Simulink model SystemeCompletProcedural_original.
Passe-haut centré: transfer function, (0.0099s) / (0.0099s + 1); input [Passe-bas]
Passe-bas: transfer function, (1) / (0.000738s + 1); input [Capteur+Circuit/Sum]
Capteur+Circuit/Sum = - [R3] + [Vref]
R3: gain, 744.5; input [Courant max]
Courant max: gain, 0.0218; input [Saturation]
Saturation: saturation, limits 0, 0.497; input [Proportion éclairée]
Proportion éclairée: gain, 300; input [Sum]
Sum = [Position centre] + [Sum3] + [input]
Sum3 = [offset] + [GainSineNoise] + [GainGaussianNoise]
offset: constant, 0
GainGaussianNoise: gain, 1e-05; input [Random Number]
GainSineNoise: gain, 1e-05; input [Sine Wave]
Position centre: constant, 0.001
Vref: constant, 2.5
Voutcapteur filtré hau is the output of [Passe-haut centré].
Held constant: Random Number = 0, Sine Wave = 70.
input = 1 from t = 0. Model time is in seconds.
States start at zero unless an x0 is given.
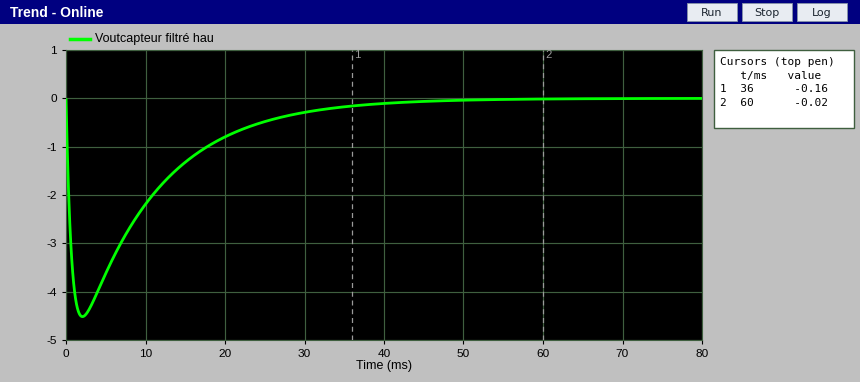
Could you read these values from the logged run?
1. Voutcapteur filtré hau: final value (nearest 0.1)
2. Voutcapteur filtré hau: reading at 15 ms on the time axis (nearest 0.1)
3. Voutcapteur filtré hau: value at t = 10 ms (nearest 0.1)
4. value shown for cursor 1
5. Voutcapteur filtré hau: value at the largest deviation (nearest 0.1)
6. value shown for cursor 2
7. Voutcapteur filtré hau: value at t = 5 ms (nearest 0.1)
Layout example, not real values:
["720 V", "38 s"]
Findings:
["0.0", "-1.3", "-2.2", "-0.16", "-4.5", "-0.02", "-3.6"]
